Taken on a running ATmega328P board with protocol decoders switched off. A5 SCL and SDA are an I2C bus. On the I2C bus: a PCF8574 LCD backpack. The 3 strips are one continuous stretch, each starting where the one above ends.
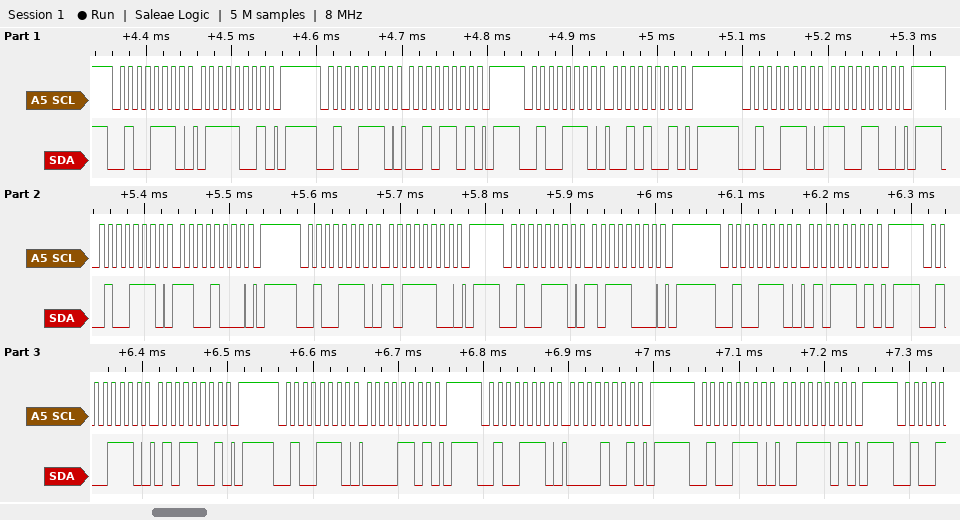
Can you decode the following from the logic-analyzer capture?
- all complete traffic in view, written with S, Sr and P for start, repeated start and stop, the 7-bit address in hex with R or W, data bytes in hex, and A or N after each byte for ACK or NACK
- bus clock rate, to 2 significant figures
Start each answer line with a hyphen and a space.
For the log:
- S 27W A 79 A P S 27W A 2D A P S 27W A 29 A P S 27W A CC A P S 27W A C8 A P S 27W A BC A P S 27W A B8 A P S 27W A 5D A P S 27W A 59 A P S 27W A 0D A P S 27W A 09 A P S 27W A 3D A P
- 100 kHz
